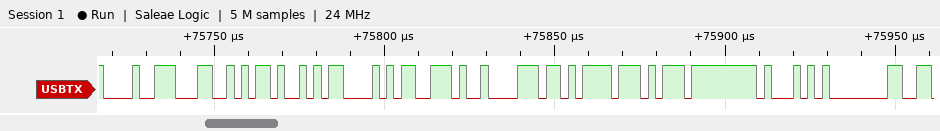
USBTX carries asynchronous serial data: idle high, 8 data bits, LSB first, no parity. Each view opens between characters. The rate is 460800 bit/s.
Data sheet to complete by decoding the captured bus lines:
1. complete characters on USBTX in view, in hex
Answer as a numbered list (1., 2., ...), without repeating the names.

1. C8, 4C, 4B, 43, 73, C2, EB, D7, FF, 51, 80
